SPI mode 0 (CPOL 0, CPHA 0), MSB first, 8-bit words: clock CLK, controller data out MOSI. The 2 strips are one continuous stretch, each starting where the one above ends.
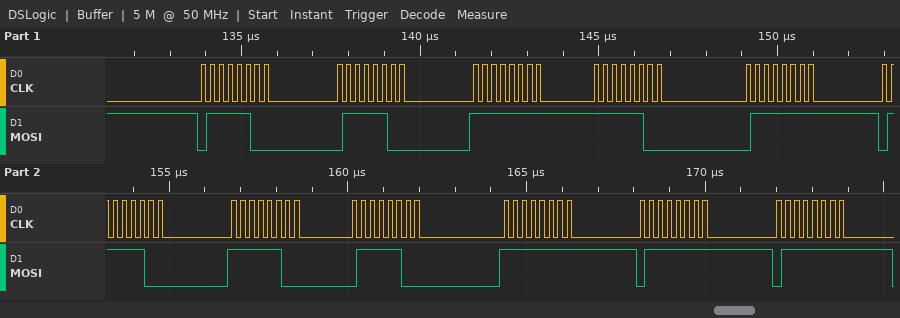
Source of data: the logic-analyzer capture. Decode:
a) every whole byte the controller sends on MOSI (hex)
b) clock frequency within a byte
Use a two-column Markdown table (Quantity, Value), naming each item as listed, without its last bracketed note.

| Quantity | Value |
|---|---|
| every whole byte the controller sends on MOSI | 0x7C 0x7C 0xFF 0xFC 0x7F 0x7C 0xFC 0x7C 0xFF 0x7F 0x7F |
| clock frequency within a byte | 4 MHz |
